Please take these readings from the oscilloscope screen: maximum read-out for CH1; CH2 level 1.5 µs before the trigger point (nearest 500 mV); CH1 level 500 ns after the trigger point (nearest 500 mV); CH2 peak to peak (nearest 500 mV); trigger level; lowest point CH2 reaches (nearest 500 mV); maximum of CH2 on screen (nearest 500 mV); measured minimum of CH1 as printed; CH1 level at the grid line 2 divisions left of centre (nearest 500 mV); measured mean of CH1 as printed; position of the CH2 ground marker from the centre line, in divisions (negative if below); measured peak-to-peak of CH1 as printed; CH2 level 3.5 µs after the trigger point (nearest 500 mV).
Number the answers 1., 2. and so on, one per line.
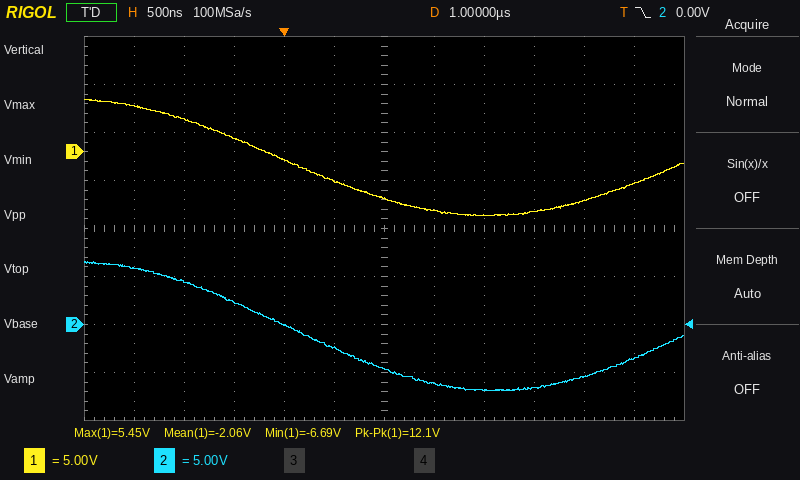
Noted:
1. 5.45 V
2. 6.0 V
3. -3.0 V
4. 13.5 V
5. 0.00 V
6. -7.0 V
7. 6.5 V
8. -6.69 V
9. -1.0 V
10. -2.06 V
11. -2.0 div
12. 12.1 V
13. -3.5 V
